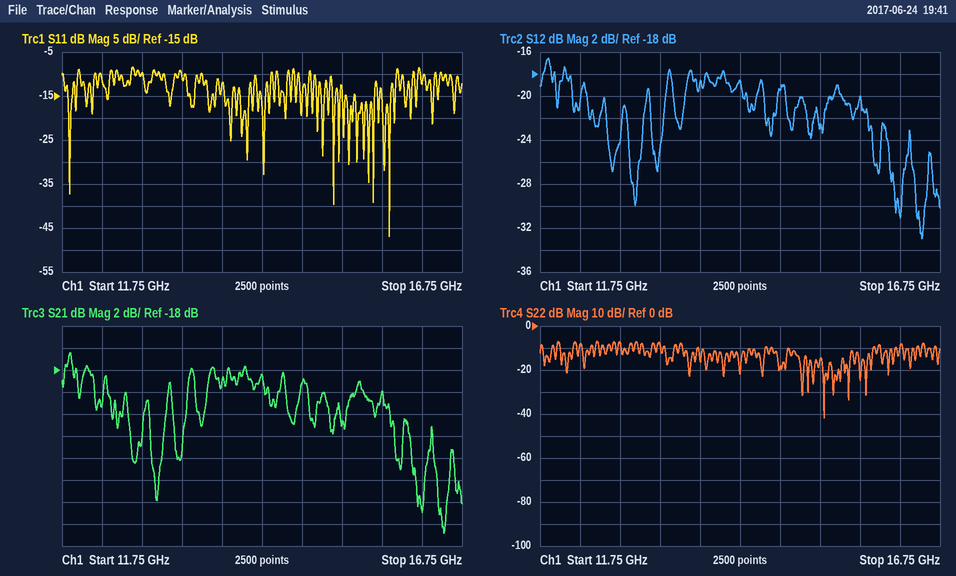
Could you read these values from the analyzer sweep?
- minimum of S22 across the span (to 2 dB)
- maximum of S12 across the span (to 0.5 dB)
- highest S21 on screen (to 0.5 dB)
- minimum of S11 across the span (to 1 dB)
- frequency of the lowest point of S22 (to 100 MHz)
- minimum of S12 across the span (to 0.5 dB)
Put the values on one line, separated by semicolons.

-42 dB; -16.5 dB; -16.5 dB; -47 dB; 15.3 GHz; -33.0 dB
